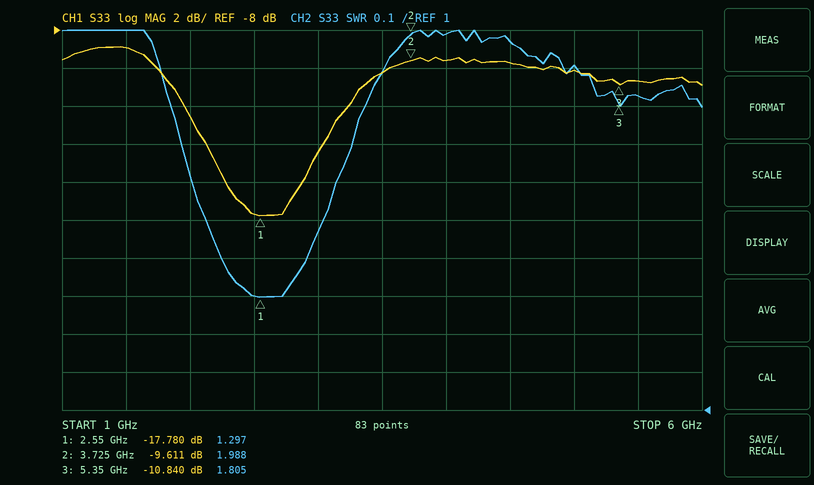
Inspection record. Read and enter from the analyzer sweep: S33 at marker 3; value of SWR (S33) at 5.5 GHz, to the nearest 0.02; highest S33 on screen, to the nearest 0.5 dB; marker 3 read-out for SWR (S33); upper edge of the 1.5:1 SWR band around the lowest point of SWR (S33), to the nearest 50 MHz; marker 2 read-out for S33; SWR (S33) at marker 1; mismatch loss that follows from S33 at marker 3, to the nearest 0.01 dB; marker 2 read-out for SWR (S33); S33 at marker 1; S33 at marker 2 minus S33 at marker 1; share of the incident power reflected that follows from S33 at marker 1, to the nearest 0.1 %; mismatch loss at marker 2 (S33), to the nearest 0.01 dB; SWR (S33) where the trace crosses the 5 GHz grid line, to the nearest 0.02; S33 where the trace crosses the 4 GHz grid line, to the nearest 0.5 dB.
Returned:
-10.840 dB
1.82
-9.0 dB
1.805
3.05 GHz
-9.611 dB
1.297
0.37 dB
1.988
-17.780 dB
8.169 dB
1.7 %
0.50 dB
1.90
-9.5 dB
